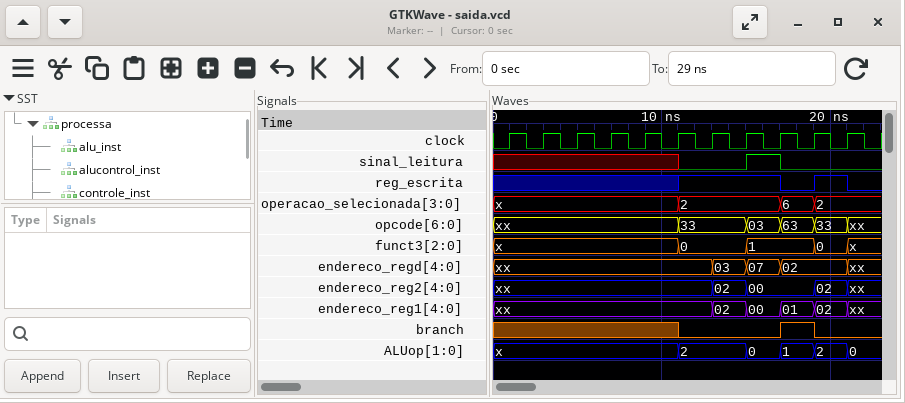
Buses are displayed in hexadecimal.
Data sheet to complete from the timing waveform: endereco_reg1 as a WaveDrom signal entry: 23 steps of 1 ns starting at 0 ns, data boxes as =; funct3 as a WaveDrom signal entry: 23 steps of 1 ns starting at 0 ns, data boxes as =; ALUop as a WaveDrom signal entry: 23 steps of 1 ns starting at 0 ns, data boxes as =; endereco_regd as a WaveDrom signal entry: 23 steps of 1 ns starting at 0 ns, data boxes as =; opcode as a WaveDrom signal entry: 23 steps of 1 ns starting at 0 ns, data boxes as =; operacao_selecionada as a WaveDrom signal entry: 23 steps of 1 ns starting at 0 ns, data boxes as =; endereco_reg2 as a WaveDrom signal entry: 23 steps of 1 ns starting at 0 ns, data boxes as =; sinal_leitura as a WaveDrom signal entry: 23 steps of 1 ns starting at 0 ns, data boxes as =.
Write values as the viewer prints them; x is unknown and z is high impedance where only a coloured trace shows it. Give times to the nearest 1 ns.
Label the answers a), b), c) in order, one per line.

a) {name: 'endereco_reg1', wave: 'x............=.=.=.=.x.', data: '02 00 01 02'}
b) {name: 'funct3', wave: 'x..........=...=...=.x.', data: '0 1 0'}
c) {name: 'ALUop', wave: 'x..........=...=.=.=.=.', data: '2 0 1 2 0'}
d) {name: 'endereco_regd', wave: 'x............=.=.=...x.', data: '03 07 02'}
e) {name: 'opcode', wave: 'x..........=...=.=.=.x.', data: '33 03 63 33'}
f) {name: 'operacao_selecionada', wave: 'x..........=.....=.=...', data: '2 6 2'}
g) {name: 'endereco_reg2', wave: 'x............=.=...=.x.', data: '02 00 02'}
h) {name: 'sinal_leitura', wave: 'x..........0...1.0.....'}
